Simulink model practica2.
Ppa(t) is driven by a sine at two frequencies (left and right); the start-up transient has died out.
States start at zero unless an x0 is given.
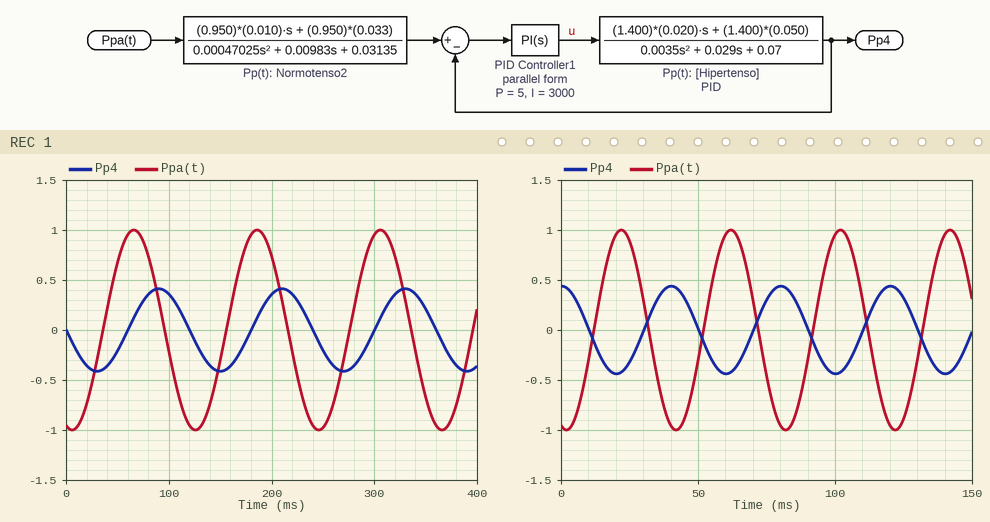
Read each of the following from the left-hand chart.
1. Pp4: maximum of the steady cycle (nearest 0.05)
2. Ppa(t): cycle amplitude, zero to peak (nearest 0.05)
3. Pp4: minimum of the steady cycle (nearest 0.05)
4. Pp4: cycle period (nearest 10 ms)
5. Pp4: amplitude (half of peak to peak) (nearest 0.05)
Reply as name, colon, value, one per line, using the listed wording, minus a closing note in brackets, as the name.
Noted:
Pp4: maximum of the steady cycle: 0.40
Ppa(t): cycle amplitude, zero to peak: 1.00
Pp4: minimum of the steady cycle: -0.40
Pp4: cycle period: 120 ms
Pp4: amplitude (half of peak to peak): 0.40
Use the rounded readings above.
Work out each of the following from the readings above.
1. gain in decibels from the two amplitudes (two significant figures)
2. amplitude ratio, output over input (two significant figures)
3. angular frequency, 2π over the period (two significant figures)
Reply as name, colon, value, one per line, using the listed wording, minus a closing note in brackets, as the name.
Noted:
gain in decibels from the two amplitudes: -8.0 dB
amplitude ratio, output over input: 0.40
angular frequency, 2π over the period: 0.052 rad/ms
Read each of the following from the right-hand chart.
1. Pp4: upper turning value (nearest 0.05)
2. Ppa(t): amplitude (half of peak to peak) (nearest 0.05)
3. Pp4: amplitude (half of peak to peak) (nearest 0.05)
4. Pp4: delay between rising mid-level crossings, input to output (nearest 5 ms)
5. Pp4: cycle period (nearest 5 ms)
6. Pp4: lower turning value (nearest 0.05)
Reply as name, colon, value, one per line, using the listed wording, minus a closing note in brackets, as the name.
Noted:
Pp4: upper turning value: 0.45
Ppa(t): amplitude (half of peak to peak): 1.00
Pp4: amplitude (half of peak to peak): 0.45
Pp4: delay between rising mid-level crossings, input to output: 20 ms
Pp4: cycle period: 40 ms
Pp4: lower turning value: -0.45
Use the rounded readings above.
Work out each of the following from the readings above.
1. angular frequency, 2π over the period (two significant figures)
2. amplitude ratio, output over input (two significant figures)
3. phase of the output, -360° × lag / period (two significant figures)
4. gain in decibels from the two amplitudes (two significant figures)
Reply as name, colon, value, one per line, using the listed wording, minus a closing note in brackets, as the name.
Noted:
angular frequency, 2π over the period: 0.16 rad/ms
amplitude ratio, output over input: 0.45
phase of the output, -360° × lag / period: -180°
gain in decibels from the two amplitudes: -6.9 dB
